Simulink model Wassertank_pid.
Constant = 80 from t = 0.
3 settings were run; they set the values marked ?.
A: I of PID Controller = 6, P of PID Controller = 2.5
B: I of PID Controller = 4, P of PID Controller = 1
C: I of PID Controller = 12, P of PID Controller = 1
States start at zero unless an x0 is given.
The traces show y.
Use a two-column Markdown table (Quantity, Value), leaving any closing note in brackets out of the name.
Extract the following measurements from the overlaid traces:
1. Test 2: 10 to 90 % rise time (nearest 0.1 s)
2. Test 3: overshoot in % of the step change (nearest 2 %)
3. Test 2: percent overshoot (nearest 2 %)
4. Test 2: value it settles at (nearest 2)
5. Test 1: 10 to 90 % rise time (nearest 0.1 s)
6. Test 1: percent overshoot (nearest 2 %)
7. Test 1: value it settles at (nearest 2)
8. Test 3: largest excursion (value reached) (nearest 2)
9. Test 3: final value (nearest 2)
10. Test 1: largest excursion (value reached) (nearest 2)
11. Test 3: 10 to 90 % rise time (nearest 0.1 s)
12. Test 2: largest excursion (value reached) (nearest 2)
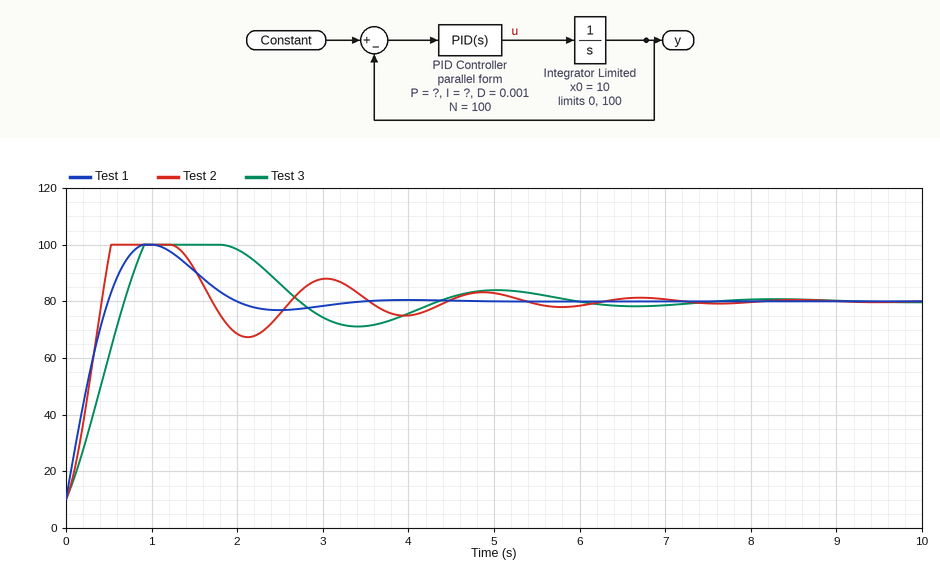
| Quantity | Value |
|---|---|
| Test 2: 10 to 90 % rise time | 0.3 s |
| Test 3: overshoot in % of the step change | 28 % |
| Test 2: percent overshoot | 28 % |
| Test 2: value it settles at | 80 |
| Test 1: 10 to 90 % rise time | 0.4 s |
| Test 1: percent overshoot | 28 % |
| Test 1: value it settles at | 80 |
| Test 3: largest excursion (value reached) | 100 |
| Test 3: final value | 80 |
| Test 1: largest excursion (value reached) | 100 |
| Test 3: 10 to 90 % rise time | 0.5 s |
| Test 2: largest excursion (value reached) | 100 |
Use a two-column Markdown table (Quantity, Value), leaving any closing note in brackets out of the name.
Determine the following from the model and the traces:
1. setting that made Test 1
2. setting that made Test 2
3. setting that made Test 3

| Quantity | Value |
|---|---|
| setting that made Test 1 | A |
| setting that made Test 2 | C |
| setting that made Test 3 | B |
